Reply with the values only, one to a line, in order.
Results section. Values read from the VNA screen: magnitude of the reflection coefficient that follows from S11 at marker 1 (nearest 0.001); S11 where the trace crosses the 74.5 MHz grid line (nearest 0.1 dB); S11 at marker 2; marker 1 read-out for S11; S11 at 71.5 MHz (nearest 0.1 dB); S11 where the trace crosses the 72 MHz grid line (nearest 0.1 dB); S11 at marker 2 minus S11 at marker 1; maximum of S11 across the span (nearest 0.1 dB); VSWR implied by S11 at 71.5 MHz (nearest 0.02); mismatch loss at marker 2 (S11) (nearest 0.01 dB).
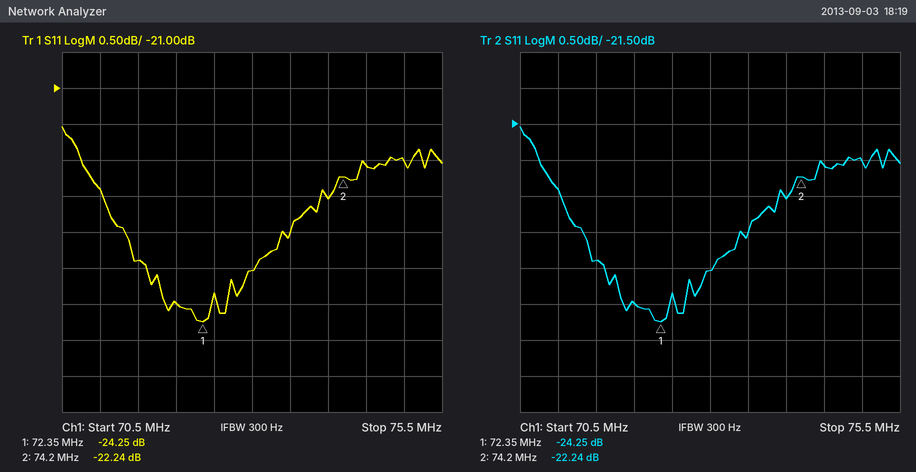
0.061
-22.1 dB
-22.24 dB
-24.25 dB
-23.4 dB
-24.0 dB
2.01 dB
-21.5 dB
1.14
0.03 dB
